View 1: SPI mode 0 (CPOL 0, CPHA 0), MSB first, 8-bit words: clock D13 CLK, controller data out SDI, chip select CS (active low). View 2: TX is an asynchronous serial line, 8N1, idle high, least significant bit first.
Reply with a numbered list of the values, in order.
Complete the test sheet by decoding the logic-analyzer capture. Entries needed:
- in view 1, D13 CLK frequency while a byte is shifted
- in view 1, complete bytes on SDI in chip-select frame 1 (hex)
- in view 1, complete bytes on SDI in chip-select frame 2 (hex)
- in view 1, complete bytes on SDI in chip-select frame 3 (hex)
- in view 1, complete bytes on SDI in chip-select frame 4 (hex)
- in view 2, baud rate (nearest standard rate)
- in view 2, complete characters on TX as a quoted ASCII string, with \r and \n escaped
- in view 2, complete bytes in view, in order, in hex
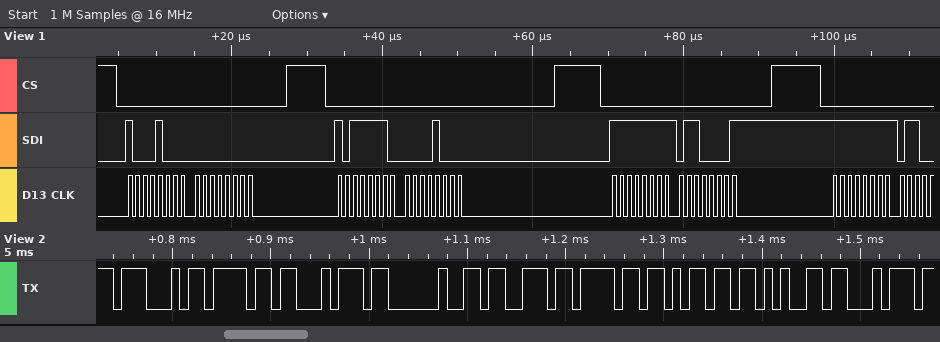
1. 1 MHz
2. 0x88 0x00
3. 0xBE 0x08
4. 0xFF 0x61
5. 0xFF
6. 115200 baud
7. "Got somet"
8. 47 6F 74 20 73 6F 6D 65 74
